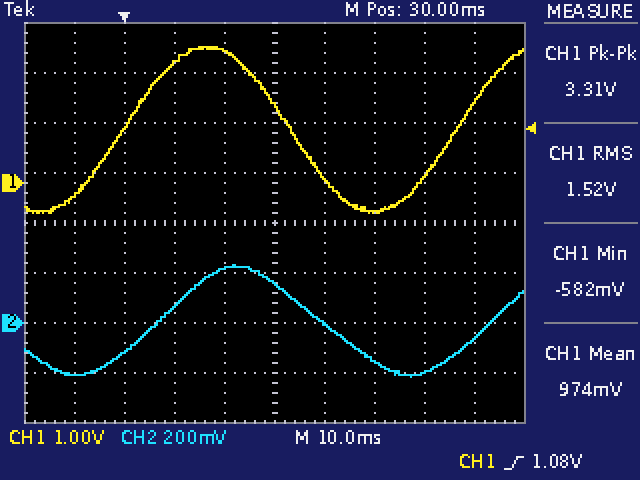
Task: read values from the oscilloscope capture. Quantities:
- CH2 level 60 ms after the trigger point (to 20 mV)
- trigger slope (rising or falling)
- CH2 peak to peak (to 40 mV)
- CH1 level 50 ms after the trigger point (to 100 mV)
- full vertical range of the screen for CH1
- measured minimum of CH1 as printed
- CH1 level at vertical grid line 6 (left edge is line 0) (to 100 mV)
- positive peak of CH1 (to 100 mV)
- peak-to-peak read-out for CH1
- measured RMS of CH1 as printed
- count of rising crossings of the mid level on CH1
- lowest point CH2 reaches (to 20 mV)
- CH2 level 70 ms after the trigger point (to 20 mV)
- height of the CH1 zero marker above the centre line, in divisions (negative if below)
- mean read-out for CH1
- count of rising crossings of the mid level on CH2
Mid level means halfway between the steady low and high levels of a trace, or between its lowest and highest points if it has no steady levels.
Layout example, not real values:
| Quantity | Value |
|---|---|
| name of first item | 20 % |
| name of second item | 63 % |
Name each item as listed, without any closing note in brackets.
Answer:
| Quantity | Value |
|---|---|
| CH2 level 60 ms after the trigger point | -200 mV |
| trigger slope | rising |
| CH2 peak to peak | 440 mV |
| CH1 level 50 ms after the trigger point | -600 mV |
| full vertical range of the screen for CH1 | 8 V |
| measured minimum of CH1 as printed | -582 mV |
| CH1 level at vertical grid line 6 (left edge is line 0) | 100 mV |
| positive peak of CH1 | 2.7 V |
| peak-to-peak read-out for CH1 | 3.31 V |
| measured RMS of CH1 as printed | 1.52 V |
| count of rising crossings of the mid level on CH1 | 2 |
| lowest point CH2 reaches | -220 mV |
| CH2 level 70 ms after the trigger point | -60 mV |
| height of the CH1 zero marker above the centre line, in divisions | +0.8 div |
| mean read-out for CH1 | 974 mV |
| count of rising crossings of the mid level on CH2 | 2 |
